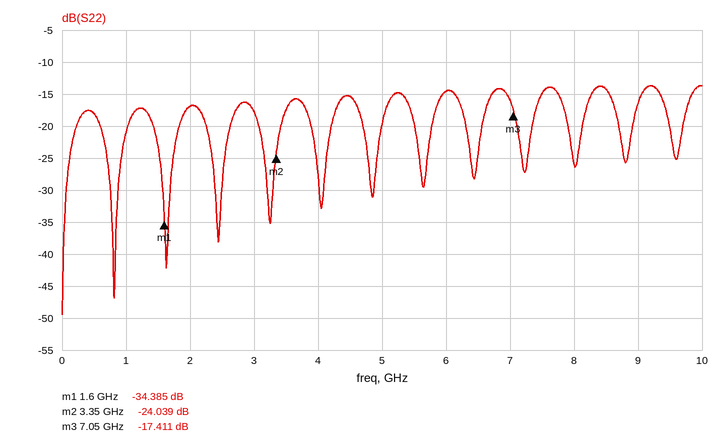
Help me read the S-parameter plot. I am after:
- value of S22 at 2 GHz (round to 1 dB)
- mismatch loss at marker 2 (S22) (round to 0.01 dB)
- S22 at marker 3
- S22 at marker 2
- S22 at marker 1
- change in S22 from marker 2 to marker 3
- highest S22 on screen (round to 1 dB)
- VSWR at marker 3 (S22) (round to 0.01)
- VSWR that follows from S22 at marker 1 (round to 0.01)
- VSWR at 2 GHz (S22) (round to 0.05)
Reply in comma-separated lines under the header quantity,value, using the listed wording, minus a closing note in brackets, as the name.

quantity,value
value of S22 at 2 GHz,-17 dB
mismatch loss at marker 2 (S22),0.02 dB
S22 at marker 3,-17.411 dB
S22 at marker 2,-24.039 dB
S22 at marker 1,-34.385 dB
change in S22 from marker 2 to marker 3,6.628 dB
highest S22 on screen,-14 dB
VSWR at marker 3 (S22),1.31
VSWR that follows from S22 at marker 1,1.04
VSWR at 2 GHz (S22),1.35
